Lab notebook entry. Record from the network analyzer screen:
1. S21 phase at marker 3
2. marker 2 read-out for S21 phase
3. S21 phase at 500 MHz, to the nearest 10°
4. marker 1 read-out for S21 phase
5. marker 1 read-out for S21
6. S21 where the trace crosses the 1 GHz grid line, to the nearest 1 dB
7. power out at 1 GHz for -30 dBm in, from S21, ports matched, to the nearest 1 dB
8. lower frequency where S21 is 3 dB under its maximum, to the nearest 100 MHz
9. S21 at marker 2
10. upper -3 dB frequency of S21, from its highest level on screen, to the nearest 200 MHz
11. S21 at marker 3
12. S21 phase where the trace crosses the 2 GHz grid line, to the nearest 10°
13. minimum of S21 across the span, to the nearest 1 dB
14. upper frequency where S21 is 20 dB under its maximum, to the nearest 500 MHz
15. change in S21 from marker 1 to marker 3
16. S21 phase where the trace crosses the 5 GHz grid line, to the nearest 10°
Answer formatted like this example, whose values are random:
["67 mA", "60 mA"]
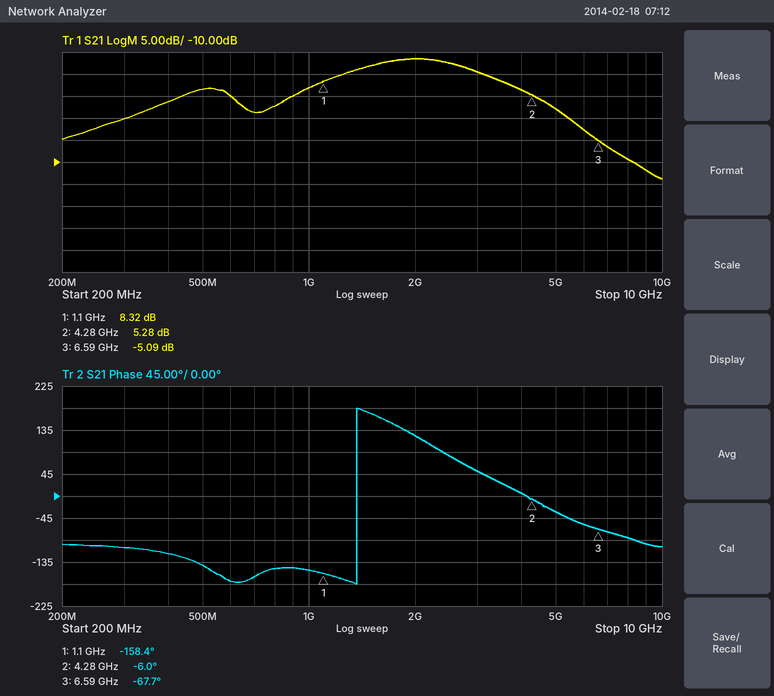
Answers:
["-67.7°", "-6.0°", "-140°", "-158.4°", "8.32 dB", "7 dB", "-23 dBm", "1.3 GHz", "5.28 dB", "3.0 GHz", "-5.09 dB", "120°", "-14 dB", "7.0 GHz", "-13.41 dB", "-30°"]
